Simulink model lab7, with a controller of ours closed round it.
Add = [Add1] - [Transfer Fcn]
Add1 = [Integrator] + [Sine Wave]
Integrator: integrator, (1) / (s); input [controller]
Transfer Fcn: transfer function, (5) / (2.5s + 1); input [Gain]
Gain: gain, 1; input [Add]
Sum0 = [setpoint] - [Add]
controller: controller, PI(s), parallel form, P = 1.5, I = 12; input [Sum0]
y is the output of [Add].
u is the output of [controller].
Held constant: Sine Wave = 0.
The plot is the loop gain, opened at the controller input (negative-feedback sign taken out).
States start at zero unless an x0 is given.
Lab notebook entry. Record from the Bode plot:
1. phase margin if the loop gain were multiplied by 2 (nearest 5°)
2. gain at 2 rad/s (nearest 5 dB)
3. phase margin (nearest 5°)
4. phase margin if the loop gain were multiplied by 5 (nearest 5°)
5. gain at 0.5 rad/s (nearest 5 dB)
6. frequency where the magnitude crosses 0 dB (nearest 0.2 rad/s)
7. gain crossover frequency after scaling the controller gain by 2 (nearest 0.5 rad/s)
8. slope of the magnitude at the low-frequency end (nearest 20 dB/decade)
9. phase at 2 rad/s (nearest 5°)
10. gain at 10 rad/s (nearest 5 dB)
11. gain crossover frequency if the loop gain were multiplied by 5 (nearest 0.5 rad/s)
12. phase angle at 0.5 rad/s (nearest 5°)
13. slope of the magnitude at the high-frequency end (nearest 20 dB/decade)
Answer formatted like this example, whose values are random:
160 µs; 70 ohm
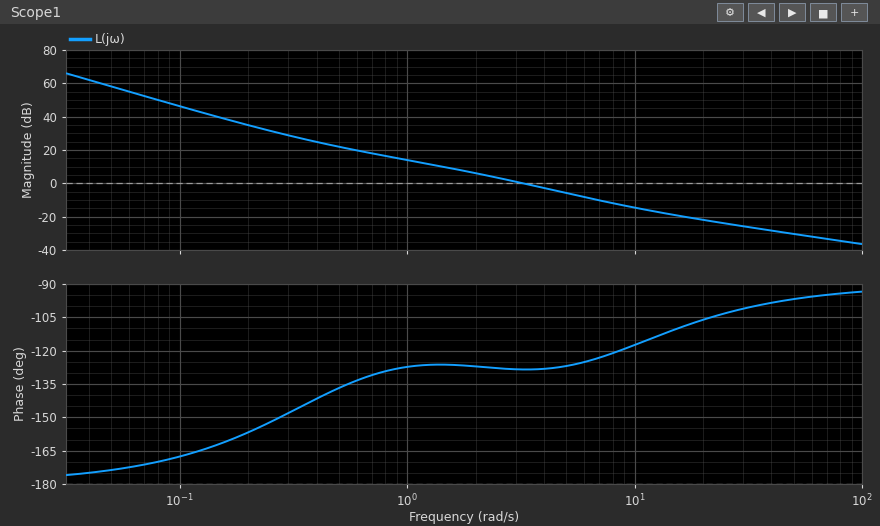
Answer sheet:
55°; 5 dB; 50°; 60°; 20 dB; 3.2 rad/s; 5.0 rad/s; -40 dB/decade; -125°; -15 dB; 9.5 rad/s; -135°; -20 dB/decade
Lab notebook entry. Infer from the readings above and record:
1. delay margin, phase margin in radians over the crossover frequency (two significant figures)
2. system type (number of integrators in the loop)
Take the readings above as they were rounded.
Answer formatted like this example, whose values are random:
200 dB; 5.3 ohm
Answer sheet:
0.27 s; 2
